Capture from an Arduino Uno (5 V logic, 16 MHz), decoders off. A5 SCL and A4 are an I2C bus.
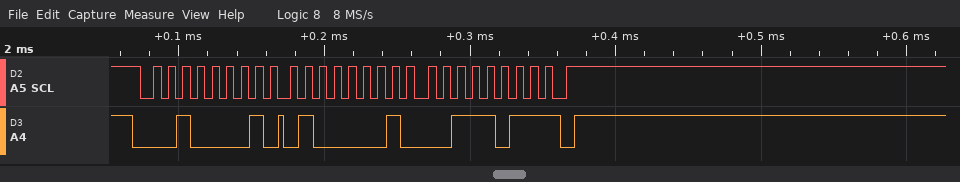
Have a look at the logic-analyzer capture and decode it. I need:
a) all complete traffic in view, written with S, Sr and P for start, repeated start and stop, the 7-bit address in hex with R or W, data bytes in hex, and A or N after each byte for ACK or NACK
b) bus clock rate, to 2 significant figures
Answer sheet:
S 10R A 41 A 3B N P
100 kHz
